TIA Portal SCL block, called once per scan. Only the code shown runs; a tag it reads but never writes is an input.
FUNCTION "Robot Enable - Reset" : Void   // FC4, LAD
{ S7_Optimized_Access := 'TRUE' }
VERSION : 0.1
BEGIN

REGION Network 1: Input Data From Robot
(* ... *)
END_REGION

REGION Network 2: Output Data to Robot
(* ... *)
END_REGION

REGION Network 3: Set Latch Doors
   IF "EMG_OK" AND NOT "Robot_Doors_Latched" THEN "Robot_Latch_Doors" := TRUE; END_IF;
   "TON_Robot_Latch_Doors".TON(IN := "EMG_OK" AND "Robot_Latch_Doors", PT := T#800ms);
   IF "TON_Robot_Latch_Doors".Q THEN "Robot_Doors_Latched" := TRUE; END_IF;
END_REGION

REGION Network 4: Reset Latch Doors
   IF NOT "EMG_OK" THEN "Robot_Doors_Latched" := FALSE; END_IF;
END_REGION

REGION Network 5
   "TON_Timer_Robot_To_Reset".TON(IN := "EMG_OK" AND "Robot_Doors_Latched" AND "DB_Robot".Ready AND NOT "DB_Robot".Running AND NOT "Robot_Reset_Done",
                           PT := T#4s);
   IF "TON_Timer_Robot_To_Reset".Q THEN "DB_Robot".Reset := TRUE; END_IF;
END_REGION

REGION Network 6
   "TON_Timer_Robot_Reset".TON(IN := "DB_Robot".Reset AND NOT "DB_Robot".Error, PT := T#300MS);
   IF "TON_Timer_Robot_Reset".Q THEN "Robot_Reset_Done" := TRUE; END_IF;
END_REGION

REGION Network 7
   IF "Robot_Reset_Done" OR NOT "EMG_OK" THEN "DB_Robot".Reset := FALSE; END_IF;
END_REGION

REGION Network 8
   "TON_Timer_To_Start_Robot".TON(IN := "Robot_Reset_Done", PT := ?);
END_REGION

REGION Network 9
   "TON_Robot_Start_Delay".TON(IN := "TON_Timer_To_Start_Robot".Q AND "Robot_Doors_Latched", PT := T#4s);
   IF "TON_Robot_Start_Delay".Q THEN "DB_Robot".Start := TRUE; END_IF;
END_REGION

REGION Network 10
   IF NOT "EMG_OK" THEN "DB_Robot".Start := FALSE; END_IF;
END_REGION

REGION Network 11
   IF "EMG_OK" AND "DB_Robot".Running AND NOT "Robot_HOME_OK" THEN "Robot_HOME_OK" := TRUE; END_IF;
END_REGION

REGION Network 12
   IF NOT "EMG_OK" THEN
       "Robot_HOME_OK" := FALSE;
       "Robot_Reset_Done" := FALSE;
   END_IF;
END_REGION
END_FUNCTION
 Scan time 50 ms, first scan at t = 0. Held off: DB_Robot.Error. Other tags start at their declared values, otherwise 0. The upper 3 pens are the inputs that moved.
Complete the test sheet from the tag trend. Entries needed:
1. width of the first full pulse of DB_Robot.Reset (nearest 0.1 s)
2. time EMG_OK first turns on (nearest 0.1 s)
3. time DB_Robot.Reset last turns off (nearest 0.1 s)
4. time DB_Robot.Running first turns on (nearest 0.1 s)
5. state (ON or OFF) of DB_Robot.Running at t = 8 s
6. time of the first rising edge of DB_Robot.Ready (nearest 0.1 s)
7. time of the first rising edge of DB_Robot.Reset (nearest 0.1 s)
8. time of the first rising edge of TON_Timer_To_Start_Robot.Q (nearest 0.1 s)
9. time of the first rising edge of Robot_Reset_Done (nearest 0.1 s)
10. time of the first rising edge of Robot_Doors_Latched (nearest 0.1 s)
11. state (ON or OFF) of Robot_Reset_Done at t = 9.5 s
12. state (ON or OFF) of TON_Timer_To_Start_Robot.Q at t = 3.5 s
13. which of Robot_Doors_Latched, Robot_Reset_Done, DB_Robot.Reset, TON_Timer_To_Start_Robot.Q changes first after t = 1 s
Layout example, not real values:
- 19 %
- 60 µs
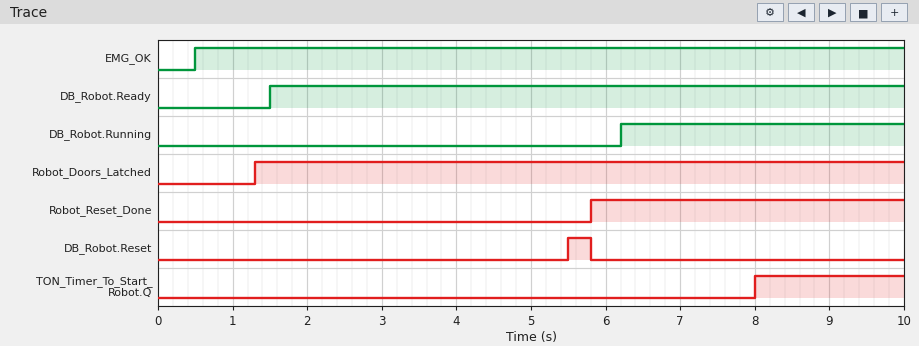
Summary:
- 0.3 s
- 0.5 s
- 5.8 s
- 6.2 s
- ON
- 1.5 s
- 5.5 s
- 8.0 s
- 5.8 s
- 1.3 s
- ON
- OFF
- Robot_Doors_Latched
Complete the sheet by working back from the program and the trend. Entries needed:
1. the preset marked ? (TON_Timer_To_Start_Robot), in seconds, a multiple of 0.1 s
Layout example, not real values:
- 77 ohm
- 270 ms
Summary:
- 2.2 s
